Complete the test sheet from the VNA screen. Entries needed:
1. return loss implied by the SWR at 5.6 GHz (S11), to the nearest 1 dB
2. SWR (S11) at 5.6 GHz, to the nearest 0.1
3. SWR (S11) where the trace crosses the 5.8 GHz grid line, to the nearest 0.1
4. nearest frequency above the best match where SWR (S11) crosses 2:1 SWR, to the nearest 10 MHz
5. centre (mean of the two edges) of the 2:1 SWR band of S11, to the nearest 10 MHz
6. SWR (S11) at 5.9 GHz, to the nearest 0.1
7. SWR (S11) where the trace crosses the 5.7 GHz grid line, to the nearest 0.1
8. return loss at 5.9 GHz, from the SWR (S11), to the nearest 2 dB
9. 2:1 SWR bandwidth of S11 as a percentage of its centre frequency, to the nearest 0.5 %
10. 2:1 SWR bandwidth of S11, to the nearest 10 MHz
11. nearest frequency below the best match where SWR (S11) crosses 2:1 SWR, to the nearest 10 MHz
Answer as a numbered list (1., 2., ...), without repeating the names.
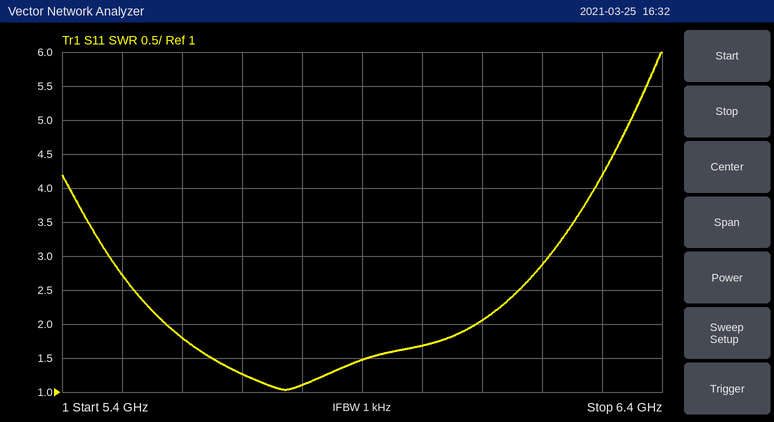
1. 11 dB
2. 1.8
3. 1.1
4. 6.09 GHz
5. 5.83 GHz
6. 1.5
7. 1.3
8. 14 dB
9. 9.0 %
10. 520 MHz
11. 5.57 GHz
